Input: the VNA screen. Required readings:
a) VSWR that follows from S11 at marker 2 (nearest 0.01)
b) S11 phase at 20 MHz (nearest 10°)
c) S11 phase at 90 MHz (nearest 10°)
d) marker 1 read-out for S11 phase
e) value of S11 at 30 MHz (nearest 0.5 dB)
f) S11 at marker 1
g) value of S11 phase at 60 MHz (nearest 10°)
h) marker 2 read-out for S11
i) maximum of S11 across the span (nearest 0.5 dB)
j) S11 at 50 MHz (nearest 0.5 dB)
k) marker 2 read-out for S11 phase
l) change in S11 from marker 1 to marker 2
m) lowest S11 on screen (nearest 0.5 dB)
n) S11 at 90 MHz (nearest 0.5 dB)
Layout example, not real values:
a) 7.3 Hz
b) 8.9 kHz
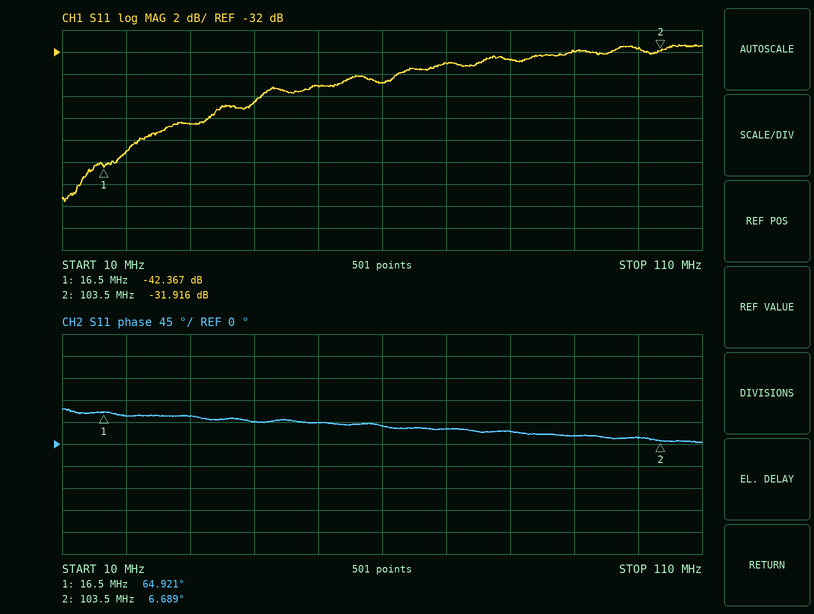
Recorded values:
a) 1.05
b) 60°
c) 20°
d) 64.921°
e) -38.5 dB
f) -42.367 dB
g) 40°
h) -31.916 dB
i) -31.5 dB
j) -35.0 dB
k) 6.689°
l) 10.451 dB
m) -45.5 dB
n) -32.0 dB
